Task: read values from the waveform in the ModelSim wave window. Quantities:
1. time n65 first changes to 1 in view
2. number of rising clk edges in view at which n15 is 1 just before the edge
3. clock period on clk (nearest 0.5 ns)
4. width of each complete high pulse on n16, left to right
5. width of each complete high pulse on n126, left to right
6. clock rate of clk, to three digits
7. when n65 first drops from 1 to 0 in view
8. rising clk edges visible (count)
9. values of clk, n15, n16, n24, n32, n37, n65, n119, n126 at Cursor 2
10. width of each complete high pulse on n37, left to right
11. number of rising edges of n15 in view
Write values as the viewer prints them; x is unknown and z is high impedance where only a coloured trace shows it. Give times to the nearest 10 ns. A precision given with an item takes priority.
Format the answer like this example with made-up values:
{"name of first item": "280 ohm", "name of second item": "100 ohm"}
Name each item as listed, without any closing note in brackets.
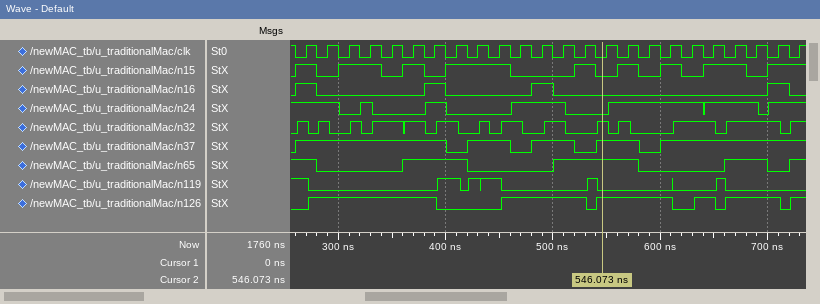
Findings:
{"time n65 first changes to 1 in view": "360 ns", "number of rising clk edges in view at which n15 is 1 just before the edge": "14", "clock period on clk": "20 ns", "width of each complete high pulse on n16, left to right": "20 ns, 20 ns, 20 ns, 20 ns", "width of each complete high pulse on n126, left to right": "120 ns, 80 ns, 70 ns, 20 ns, 50 ns", "clock rate of clk, to three digits": "50.0 MHz", "when n65 first drops from 1 to 0 in view": "280 ns", "rising clk edges visible": "24", "values of clk, n15, n16, n24, n32, n37, n65, n119, n126 at Cursor 2": "clk=0, n15=0, n16=0, n24=0, n32=1, n37=1, n65=1, n119=0, n126=1", "width of each complete high pulse on n37, left to right": "140 ns, 40 ns, 40 ns, 40 ns", "number of rising edges of n15 in view": "9"}
